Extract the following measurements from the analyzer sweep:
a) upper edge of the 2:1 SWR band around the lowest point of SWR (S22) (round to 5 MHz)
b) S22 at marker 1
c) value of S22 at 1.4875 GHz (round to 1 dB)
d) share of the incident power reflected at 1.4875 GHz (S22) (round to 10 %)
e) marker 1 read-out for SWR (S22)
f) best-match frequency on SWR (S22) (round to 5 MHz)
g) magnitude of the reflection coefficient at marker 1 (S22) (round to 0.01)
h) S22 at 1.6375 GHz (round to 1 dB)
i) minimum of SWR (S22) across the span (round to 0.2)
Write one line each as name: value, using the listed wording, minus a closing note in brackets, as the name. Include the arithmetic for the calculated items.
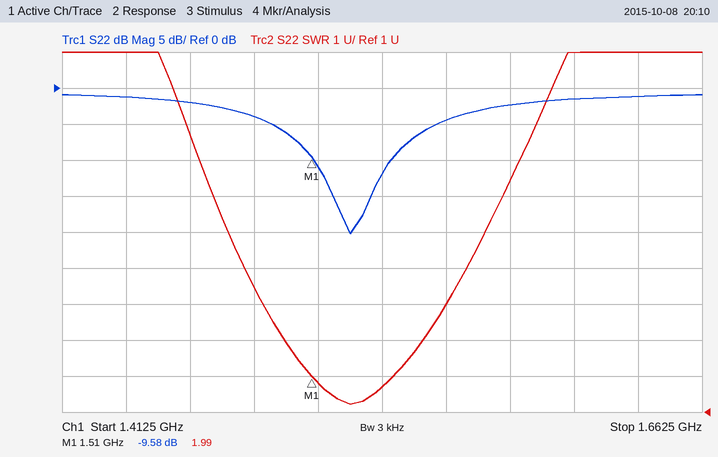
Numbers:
upper edge of the 2:1 SWR band around the lowest point of SWR (S22): 1.540 GHz
S22 at marker 1: -9.58 dB
value of S22 at 1.4875 GHz: -4 dB
share of the incident power reflected at 1.4875 GHz (S22): 10^(-4/10) ≈ 40 %
marker 1 read-out for SWR: 1.99
best-match frequency on SWR (S22): 1.525 GHz
magnitude of the reflection coefficient at marker 1 (S22): 10^(-9.58/20) ≈ 0.33
S22 at 1.6375 GHz: -1 dB
minimum of SWR (S22) across the span: 1.2
